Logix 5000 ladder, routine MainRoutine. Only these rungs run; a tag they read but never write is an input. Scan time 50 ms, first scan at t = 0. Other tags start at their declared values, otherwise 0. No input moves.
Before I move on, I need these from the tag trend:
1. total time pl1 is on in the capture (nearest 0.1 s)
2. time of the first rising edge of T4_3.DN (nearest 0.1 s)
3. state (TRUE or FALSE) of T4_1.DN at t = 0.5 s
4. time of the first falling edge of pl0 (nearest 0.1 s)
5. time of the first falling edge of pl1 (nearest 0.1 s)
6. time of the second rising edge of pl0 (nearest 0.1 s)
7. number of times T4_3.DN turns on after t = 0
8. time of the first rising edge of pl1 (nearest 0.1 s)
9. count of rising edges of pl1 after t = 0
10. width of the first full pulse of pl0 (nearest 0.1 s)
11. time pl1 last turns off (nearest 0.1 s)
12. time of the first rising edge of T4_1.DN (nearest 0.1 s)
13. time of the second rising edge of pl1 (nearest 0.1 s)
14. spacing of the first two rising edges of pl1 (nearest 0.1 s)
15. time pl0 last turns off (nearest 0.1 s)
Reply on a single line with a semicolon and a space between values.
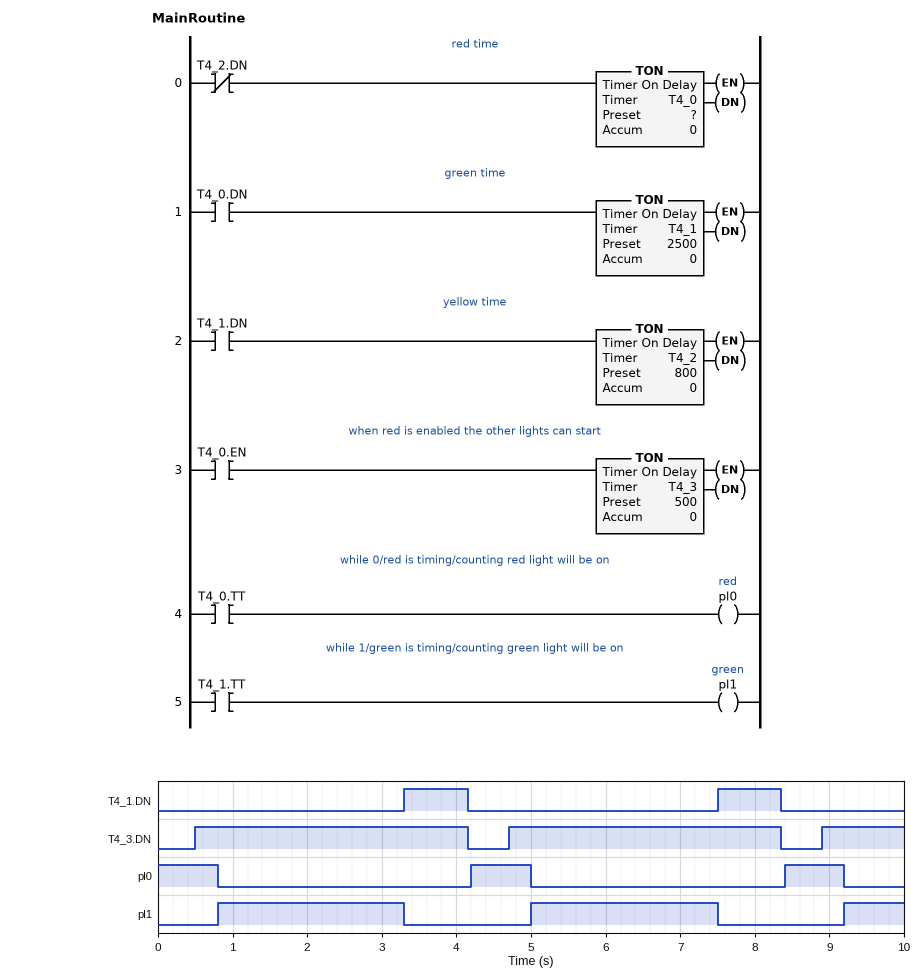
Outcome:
5.8 s; 0.5 s; FALSE; 0.8 s; 3.3 s; 8.4 s; 3; 0.8 s; 3; 0.8 s; 7.5 s; 3.3 s; 5.0 s; 4.2 s; 9.2 s
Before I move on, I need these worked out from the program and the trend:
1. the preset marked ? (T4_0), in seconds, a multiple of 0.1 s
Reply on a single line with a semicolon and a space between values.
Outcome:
0.8 s
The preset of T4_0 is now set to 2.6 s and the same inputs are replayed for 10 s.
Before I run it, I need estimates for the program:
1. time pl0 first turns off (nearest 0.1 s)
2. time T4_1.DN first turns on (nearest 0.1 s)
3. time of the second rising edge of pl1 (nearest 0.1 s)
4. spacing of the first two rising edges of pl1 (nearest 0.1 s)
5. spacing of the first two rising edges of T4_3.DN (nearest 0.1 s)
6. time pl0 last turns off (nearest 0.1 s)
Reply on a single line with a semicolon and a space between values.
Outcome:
2.6 s; 5.1 s; 8.6 s; 6.0 s; 6.0 s; 8.6 s
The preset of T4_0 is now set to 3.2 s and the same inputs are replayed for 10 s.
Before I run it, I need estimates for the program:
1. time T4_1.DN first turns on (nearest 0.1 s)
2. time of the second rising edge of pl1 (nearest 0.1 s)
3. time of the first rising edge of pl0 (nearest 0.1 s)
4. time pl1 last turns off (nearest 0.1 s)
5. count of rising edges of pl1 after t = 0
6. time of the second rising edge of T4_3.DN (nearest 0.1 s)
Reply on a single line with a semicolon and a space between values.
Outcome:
5.7 s; 9.8 s; 6.6 s; 5.7 s; 2; 7.1 s
